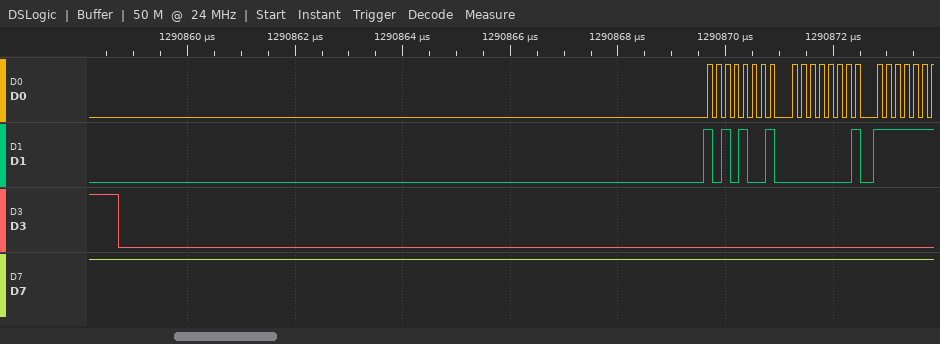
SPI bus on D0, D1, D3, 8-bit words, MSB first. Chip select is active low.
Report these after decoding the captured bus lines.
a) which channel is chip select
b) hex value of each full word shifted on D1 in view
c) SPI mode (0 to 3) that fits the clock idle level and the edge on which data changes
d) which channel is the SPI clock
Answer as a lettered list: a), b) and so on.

a) D3
b) A9, 01
c) 0
d) D0
